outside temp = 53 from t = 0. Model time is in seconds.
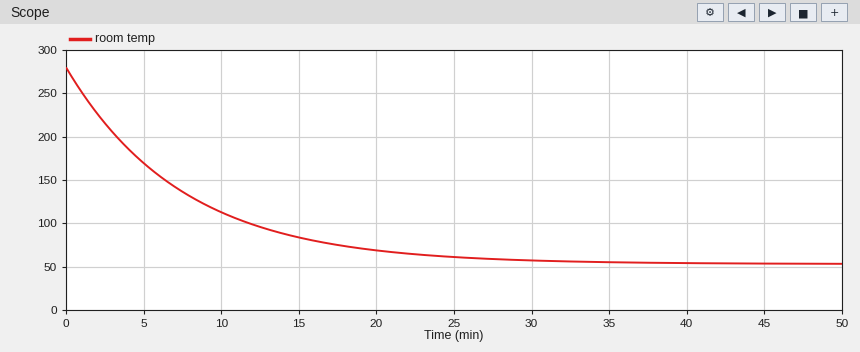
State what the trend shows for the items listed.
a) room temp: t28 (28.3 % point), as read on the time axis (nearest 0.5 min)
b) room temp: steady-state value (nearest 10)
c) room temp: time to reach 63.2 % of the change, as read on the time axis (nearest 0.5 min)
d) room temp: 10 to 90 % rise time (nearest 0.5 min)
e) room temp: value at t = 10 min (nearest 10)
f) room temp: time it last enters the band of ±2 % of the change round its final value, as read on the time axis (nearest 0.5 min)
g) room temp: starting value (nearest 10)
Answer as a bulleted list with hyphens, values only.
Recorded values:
- 2.5 min
- 50
- 7.5 min
- 16.5 min
- 110
- 29.5 min
- 280
